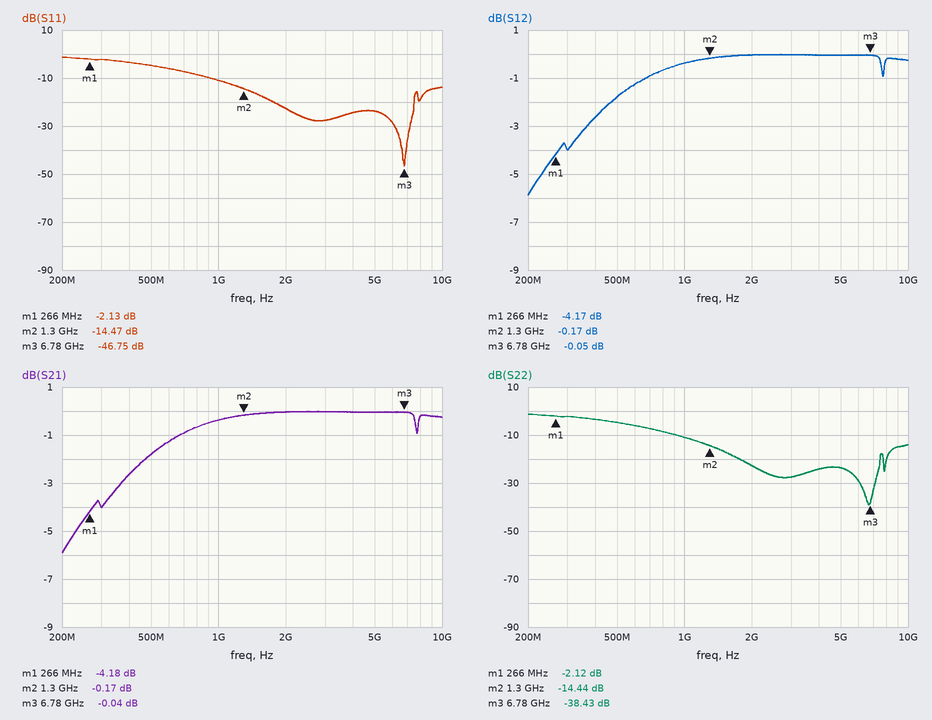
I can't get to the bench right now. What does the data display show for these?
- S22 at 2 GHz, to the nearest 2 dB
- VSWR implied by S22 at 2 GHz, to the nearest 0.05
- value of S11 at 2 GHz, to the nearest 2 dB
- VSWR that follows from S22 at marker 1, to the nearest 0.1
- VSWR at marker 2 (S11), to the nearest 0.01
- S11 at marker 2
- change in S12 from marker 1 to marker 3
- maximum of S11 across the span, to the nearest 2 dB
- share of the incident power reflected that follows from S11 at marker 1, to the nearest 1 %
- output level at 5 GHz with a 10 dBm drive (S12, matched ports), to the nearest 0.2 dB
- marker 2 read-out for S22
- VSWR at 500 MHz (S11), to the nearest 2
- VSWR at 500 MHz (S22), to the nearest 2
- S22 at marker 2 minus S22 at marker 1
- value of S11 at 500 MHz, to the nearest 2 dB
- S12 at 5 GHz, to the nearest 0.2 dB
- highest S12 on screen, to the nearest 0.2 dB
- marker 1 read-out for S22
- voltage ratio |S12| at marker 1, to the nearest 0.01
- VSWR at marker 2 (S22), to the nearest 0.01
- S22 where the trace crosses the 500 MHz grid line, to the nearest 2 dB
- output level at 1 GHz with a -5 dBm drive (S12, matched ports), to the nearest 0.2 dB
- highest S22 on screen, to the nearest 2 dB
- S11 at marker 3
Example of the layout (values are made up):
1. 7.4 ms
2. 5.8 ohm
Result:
1. -22 dB
2. 1.15
3. -22 dB
4. 8.2
5. 1.47
6. -14.47 dB
7. 4.12 dB
8. -2 dB
9. 61 %
10. 10.0 dBm
11. -14.44 dB
12. 4
13. 4
14. -12.32 dB
15. -4 dB
16. 0.0 dB
17. 0.0 dB
18. -2.12 dB
19. 0.62
20. 1.47
21. -4 dB
22. -5.4 dBm
23. -2 dB
24. -46.75 dB
